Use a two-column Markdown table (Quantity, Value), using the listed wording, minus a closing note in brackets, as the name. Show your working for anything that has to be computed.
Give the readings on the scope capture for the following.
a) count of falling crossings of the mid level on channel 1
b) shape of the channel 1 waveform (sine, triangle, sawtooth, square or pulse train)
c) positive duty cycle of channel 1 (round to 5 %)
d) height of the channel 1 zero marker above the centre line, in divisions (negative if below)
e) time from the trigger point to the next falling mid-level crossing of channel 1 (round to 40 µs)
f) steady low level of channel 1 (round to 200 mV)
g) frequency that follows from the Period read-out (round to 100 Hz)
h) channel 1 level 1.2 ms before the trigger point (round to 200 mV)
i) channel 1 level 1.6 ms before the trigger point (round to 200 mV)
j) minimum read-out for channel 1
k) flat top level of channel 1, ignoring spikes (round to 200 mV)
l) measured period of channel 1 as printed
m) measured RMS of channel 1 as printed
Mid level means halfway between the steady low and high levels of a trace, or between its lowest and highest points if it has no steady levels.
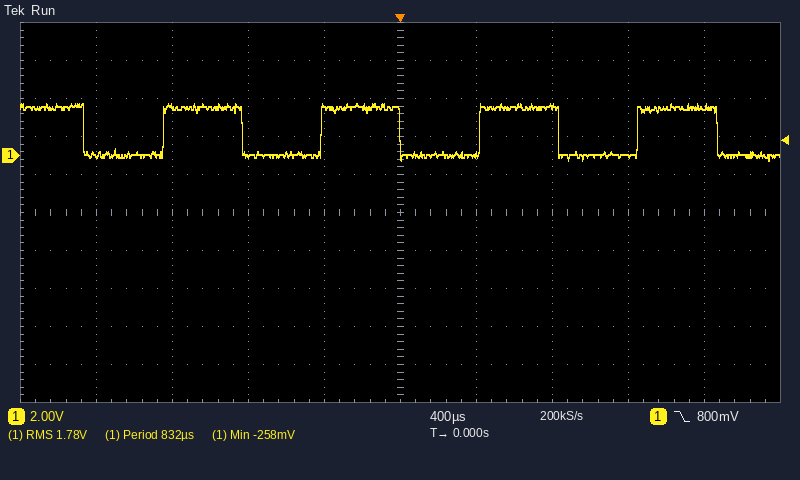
| Quantity | Value |
|---|---|
| count of falling crossings of the mid level on channel 1 | 5 |
| shape of the channel 1 waveform | square |
| positive duty cycle of channel 1 | 50 % |
| height of the channel 1 zero marker above the centre line, in divisions | +1.5 div |
| time from the trigger point to the next falling mid-level crossing of channel 1 | 840 µs |
| steady low level of channel 1 | 0.0 V |
| frequency that follows from the Period read-out | 1 / 832 µs ≈ 1.2 kHz |
| channel 1 level 1.2 ms before the trigger point | 2.6 V |
| channel 1 level 1.6 ms before the trigger point | 0.0 V |
| minimum read-out for channel 1 | -258 mV |
| flat top level of channel 1, ignoring spikes | 2.6 V |
| measured period of channel 1 as printed | 832 µs |
| measured RMS of channel 1 as printed | 1.78 V |
